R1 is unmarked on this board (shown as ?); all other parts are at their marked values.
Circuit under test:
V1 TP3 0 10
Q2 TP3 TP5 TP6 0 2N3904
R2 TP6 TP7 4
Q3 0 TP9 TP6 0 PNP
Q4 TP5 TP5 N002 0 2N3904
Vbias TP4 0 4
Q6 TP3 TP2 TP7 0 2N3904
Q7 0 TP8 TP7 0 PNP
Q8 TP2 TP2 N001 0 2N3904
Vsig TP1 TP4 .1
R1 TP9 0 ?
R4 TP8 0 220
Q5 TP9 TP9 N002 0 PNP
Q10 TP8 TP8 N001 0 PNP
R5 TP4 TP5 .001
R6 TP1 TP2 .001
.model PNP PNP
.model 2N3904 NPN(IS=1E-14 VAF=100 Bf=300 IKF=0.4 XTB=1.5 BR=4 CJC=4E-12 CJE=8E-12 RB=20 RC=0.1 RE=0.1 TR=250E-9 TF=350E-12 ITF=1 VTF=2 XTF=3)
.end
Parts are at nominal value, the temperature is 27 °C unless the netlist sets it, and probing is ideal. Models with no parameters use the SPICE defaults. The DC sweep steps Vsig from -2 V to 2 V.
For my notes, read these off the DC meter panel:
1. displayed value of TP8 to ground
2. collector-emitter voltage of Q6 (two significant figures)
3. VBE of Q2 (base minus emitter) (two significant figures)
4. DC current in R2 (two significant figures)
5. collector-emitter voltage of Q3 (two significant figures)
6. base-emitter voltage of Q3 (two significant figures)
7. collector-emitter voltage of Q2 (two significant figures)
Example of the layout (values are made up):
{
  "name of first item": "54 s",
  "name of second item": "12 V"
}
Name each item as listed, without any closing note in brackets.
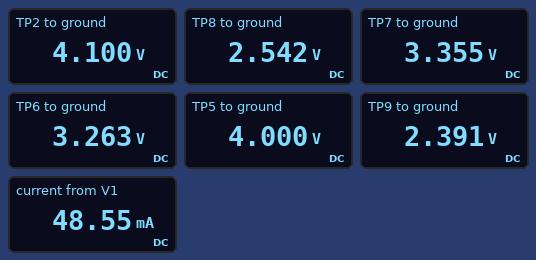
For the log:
{
  "displayed value of TP8 to ground": "2.542 V",
  "collector-emitter voltage of Q6": "6.6 V",
  "VBE of Q2 (base minus emitter)": "740 mV",
  "DC current in R2": "23 mA",
  "collector-emitter voltage of Q3": "-3.3 V",
  "base-emitter voltage of Q3": "-870 mV",
  "collector-emitter voltage of Q2": "6.7 V"
}
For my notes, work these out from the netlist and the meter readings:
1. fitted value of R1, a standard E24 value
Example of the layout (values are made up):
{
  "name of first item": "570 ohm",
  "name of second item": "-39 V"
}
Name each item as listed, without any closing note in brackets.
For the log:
{
  "fitted value of R1, a standard E24 value": "82 Ω"
}
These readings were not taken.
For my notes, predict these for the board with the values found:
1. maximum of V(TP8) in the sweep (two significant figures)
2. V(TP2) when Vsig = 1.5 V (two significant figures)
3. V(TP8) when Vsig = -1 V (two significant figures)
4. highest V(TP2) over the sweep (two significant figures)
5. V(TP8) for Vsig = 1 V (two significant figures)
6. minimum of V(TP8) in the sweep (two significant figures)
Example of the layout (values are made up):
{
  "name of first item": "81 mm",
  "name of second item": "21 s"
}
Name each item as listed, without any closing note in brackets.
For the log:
{
  "maximum of V(TP8) in the sweep": "4.4 V",
  "V(TP2) when Vsig = 1.5 V": "5.5 V",
  "V(TP8) when Vsig = -1 V": "1.5 V",
  "highest V(TP2) over the sweep": "6.0 V",
  "V(TP8) for Vsig = 1 V": "3.4 V",
  "minimum of V(TP8) in the sweep": "770 mV"
}
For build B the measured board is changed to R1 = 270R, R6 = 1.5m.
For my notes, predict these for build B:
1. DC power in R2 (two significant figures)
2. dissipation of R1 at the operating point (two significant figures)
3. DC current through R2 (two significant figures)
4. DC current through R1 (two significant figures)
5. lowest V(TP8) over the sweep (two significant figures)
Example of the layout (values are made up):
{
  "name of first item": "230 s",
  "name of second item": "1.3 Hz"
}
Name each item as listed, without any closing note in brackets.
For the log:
{
  "DC power in R2": "830 µW",
  "dissipation of R1 at the operating point": "22 mW",
  "DC current through R2": "14 mA",
  "DC current through R1": "9.1 mA",
  "lowest V(TP8) over the sweep": "770 mV"
}
